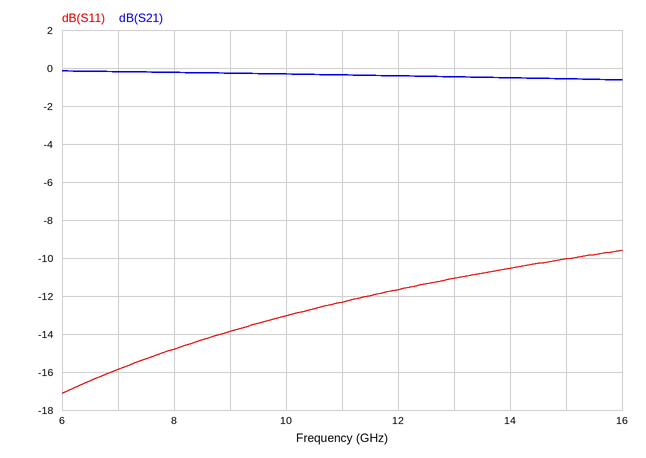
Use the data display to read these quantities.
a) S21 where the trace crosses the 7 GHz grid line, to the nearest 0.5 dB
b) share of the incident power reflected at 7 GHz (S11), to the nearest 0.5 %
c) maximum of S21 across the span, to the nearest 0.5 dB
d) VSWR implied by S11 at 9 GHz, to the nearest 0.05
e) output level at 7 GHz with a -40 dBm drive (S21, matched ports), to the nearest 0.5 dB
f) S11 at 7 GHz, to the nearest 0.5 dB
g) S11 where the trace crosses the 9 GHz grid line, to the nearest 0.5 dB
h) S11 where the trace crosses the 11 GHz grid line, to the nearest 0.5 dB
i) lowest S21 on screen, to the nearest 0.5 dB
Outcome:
0.0 dB
2.5 %
0.0 dB
1.50
-40.0 dBm
-16.0 dB
-14.0 dB
-12.5 dB
-0.5 dB
